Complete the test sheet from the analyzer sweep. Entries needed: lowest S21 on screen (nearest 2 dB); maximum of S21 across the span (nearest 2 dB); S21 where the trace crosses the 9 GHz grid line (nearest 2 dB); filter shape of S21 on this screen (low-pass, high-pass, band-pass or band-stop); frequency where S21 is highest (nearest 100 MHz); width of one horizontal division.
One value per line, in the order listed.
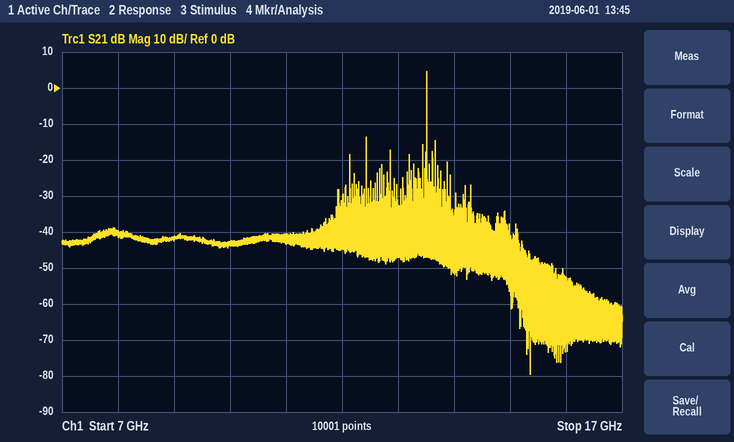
-80 dB
4 dB
-42 dB
band-pass
13.5 GHz
1 GHz
